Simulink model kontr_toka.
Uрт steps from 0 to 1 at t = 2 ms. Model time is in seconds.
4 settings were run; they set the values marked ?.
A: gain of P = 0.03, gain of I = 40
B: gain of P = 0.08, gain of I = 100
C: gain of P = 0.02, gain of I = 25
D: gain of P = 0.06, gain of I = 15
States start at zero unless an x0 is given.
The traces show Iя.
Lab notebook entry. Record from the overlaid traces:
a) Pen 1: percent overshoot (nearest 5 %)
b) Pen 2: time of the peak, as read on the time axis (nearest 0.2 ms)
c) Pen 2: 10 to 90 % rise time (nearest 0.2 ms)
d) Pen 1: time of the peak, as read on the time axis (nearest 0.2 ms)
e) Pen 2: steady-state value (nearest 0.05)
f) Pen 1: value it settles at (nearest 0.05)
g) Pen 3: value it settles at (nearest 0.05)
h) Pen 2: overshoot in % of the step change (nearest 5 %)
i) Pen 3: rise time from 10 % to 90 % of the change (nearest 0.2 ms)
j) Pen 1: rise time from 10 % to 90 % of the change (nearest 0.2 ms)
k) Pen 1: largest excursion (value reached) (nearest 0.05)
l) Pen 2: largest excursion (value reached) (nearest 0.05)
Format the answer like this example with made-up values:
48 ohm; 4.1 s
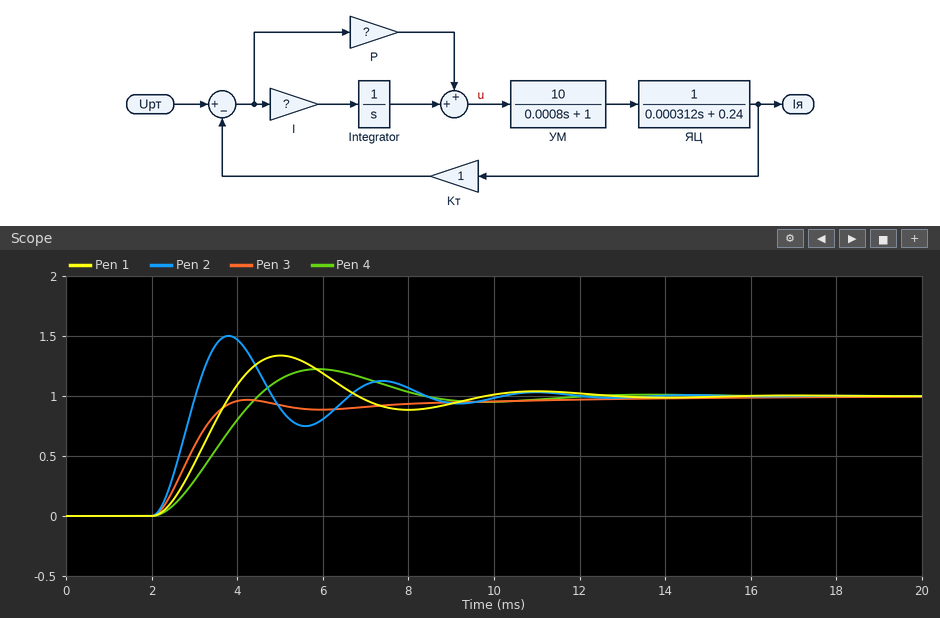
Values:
35 %; 3.8 ms; 0.6 ms; 5.0 ms; 1.00; 1.00; 1.00; 50 %; 1.4 ms; 1.2 ms; 1.35; 1.50
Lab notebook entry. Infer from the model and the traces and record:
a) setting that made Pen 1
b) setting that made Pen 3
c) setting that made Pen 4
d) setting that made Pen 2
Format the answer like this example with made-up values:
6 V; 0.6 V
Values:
A; D; C; B
